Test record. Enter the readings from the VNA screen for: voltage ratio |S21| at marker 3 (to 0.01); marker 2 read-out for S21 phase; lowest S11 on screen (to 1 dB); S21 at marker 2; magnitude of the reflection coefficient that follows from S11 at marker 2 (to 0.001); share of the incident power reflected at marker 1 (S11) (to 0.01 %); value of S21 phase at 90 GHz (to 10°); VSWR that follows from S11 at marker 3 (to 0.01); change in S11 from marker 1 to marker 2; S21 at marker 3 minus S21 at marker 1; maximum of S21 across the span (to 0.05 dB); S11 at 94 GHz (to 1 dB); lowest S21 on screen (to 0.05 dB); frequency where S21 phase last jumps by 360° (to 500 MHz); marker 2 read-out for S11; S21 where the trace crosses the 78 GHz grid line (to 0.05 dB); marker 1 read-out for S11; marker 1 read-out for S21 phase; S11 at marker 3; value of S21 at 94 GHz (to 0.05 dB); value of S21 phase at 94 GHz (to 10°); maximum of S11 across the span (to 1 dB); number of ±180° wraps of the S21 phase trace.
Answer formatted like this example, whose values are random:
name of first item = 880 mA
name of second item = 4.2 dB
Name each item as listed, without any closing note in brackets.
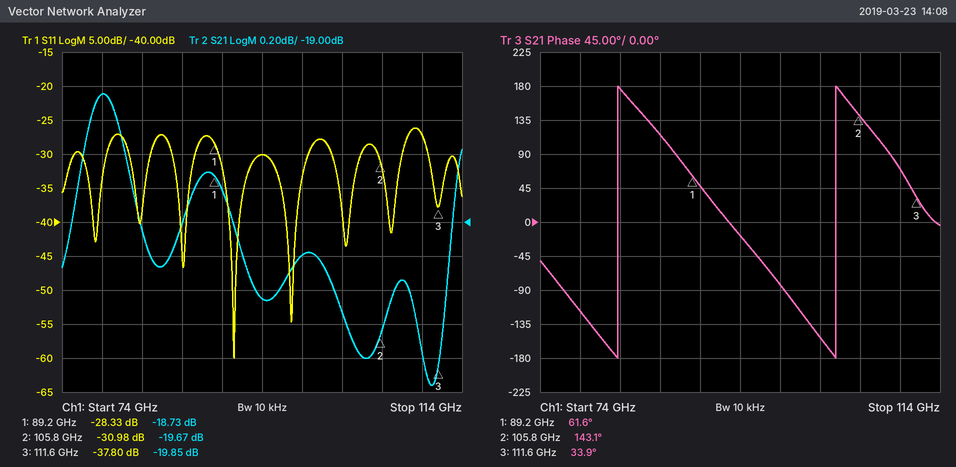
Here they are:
voltage ratio |S21| at marker 3 = 0.10
marker 2 read-out for S21 phase = 143.1°
lowest S11 on screen = -60 dB
S21 at marker 2 = -19.67 dB
magnitude of the reflection coefficient that follows from S11 at marker 2 = 0.028
share of the incident power reflected at marker 1 (S11) = 0.15 %
value of S21 phase at 90 GHz = 50°
VSWR that follows from S11 at marker 3 = 1.03
change in S11 from marker 1 to marker 2 = -2.65 dB
S21 at marker 3 minus S21 at marker 1 = -1.12 dB
maximum of S21 across the span = -18.25 dB
S11 at 94 GHz = -30 dB
lowest S21 on screen = -19.95 dB
frequency where S21 phase last jumps by 360° = 103.5 GHz
marker 2 read-out for S11 = -30.98 dB
S21 where the trace crosses the 78 GHz grid line = -18.25 dB
marker 1 read-out for S11 = -28.33 dB
marker 1 read-out for S21 phase = 61.6°
S11 at marker 3 = -37.80 dB
value of S21 at 94 GHz = -19.45 dB
value of S21 phase at 94 GHz = -20°
maximum of S11 across the span = -26 dB
number of ±180° wraps of the S21 phase trace = 2
